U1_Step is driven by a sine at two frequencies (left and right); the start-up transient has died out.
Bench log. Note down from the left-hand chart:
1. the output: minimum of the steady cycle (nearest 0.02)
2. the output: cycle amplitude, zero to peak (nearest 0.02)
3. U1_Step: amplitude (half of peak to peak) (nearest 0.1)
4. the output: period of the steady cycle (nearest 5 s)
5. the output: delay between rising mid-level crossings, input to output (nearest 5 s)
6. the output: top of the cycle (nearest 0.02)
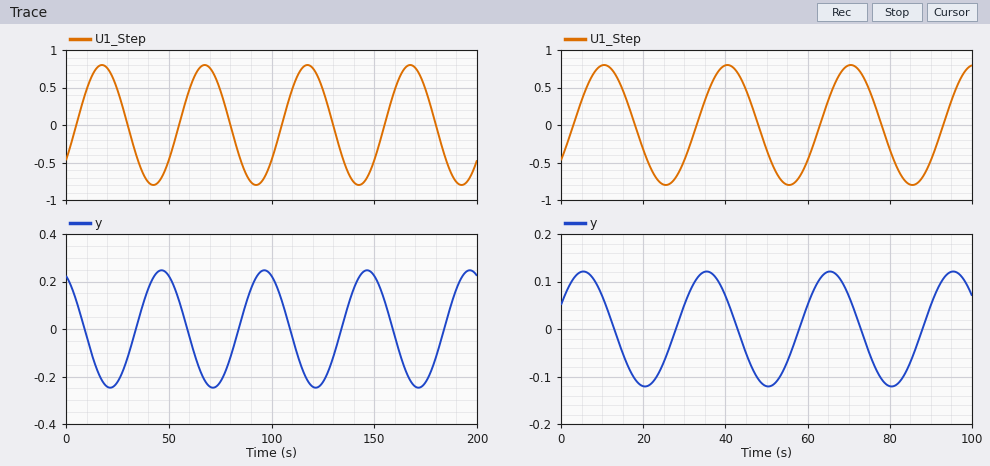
-0.24
0.24
0.8
50 s
30 s
0.24
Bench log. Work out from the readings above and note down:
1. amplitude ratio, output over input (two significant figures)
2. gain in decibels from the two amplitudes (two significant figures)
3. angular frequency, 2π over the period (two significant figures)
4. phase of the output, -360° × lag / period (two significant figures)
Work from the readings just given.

0.30
-10 dB
0.13 rad/s
-220°
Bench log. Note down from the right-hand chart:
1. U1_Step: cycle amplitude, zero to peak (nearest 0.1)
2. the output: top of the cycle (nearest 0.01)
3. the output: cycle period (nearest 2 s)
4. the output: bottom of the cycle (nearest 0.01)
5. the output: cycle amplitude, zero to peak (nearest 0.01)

0.8
0.12
30 s
-0.12
0.12
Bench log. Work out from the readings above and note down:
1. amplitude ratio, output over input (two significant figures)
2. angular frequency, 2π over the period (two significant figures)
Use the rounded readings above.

0.15
0.21 rad/s
